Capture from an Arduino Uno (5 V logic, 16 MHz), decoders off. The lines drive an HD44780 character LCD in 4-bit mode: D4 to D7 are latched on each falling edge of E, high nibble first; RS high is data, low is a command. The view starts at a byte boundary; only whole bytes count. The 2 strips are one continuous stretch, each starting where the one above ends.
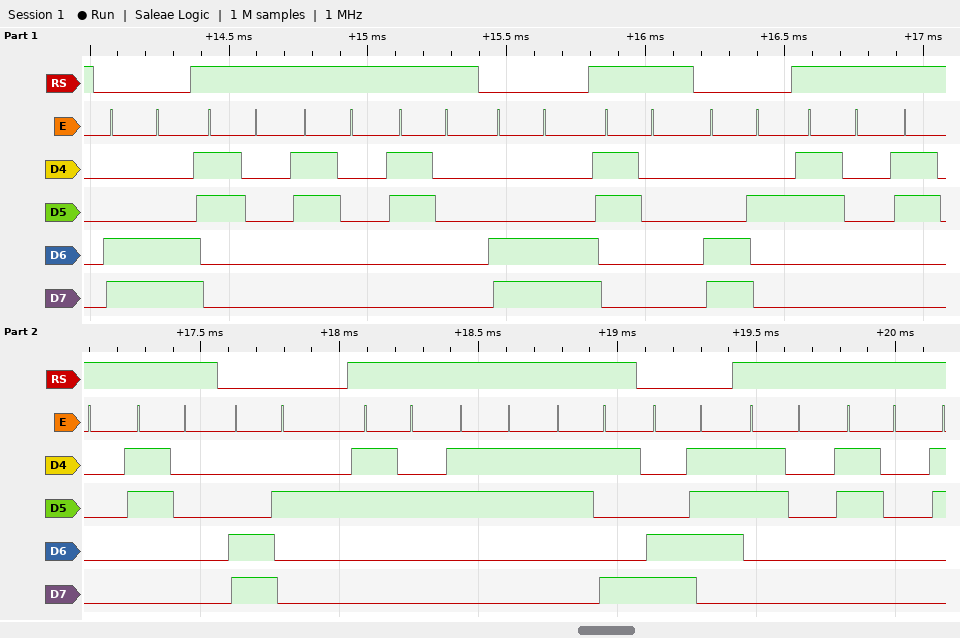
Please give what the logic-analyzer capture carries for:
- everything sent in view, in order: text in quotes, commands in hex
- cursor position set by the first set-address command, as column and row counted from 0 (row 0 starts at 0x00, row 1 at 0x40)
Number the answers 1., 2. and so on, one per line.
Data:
1. 0xCC "000" 0xCC "0" 0xC2 "000" 0xC2 "239" 0xC7 "00"
2. column 12, row 1
